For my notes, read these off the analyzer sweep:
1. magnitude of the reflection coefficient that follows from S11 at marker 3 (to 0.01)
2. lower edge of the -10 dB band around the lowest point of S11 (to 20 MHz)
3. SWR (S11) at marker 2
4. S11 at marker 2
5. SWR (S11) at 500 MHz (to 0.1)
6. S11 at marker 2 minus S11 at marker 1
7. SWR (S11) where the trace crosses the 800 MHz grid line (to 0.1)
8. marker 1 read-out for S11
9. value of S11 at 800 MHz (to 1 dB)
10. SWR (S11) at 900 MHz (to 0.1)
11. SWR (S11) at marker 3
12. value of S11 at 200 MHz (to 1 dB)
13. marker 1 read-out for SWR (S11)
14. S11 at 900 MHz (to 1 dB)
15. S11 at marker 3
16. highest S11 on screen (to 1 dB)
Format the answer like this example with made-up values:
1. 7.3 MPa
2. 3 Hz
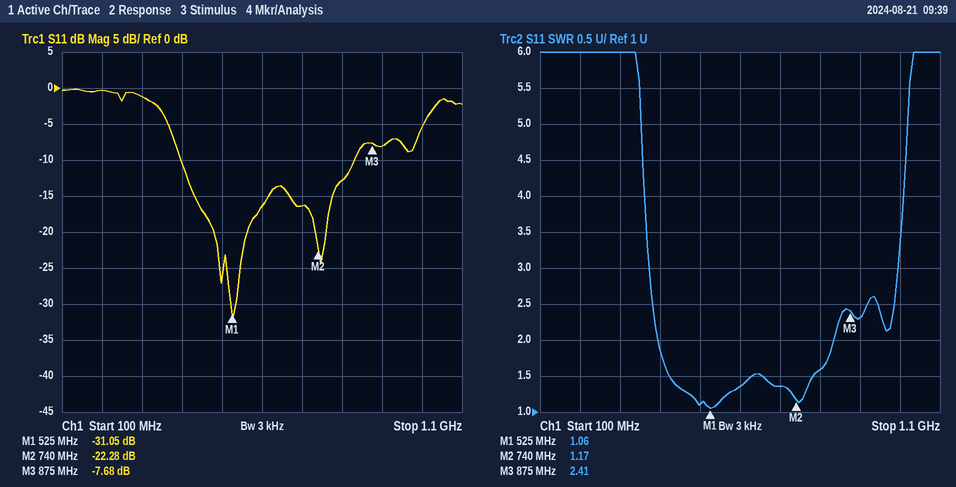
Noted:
1. 0.41
2. 400 MHz
3. 1.17
4. -22.28 dB
5. 1.1
6. 8.77 dB
7. 1.6
8. -31.05 dB
9. -13 dB
10. 2.3
11. 2.41
12. 0 dB
13. 1.06
14. -8 dB
15. -7.68 dB
16. 0 dB
